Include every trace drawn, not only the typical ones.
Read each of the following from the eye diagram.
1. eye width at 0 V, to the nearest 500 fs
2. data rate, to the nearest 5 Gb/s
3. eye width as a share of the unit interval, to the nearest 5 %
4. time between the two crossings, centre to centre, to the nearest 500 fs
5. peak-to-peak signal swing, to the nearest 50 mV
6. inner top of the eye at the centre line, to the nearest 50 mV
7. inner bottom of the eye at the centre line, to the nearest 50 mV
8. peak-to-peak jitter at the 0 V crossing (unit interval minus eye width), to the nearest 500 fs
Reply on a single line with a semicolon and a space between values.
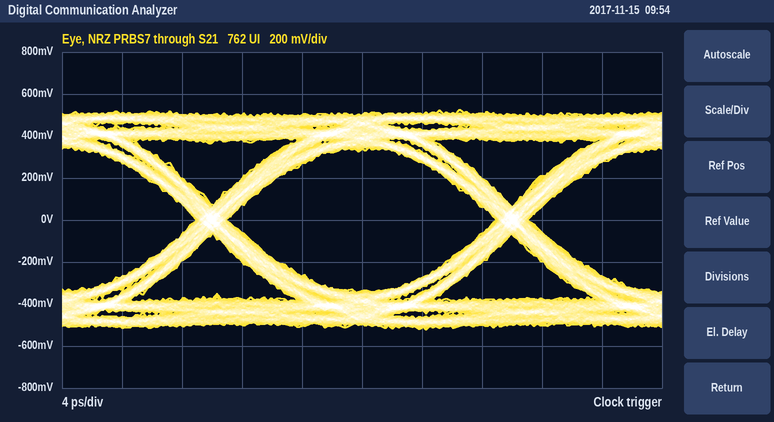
18.0 ps; 50 Gb/s; 90 %; 20.0 ps; 1.05 V; 350 mV; -350 mV; 2.0 ps
